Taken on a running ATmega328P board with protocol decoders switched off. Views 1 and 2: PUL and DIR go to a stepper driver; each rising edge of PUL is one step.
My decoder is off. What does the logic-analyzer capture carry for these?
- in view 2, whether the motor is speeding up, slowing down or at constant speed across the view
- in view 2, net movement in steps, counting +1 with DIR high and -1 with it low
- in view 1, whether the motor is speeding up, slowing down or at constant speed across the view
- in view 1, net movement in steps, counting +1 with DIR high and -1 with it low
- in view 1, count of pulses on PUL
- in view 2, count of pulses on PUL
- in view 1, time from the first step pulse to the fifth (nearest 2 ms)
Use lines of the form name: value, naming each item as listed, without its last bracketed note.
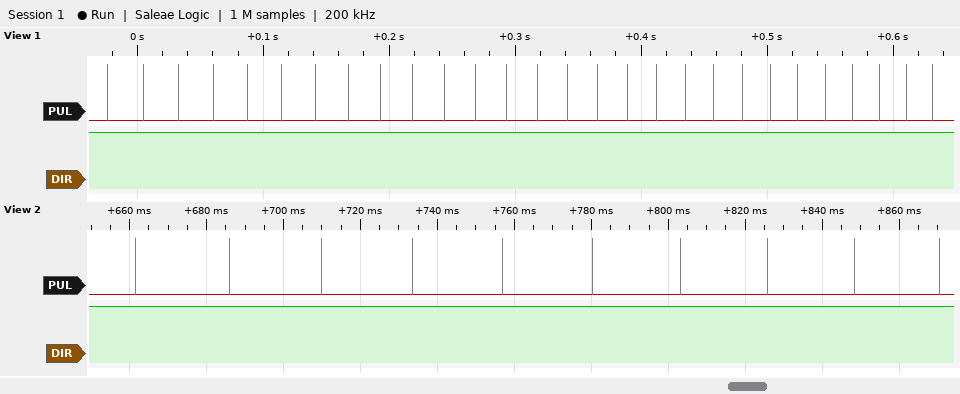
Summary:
in view 2, whether the motor is speeding up, slowing down or at constant speed across the view: speeding up
in view 2, net movement in steps, counting +1 with DIR high and -1 with it low: +10
in view 1, whether the motor is speeding up, slowing down or at constant speed across the view: speeding up
in view 1, net movement in steps, counting +1 with DIR high and -1 with it low: +28
in view 1, count of pulses on PUL: 28
in view 2, count of pulses on PUL: 10
in view 1, time from the first step pulse to the fifth: 112 ms
